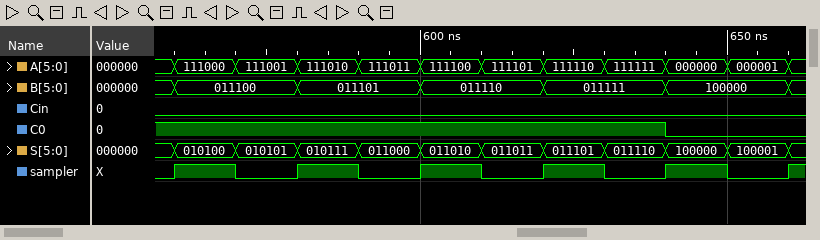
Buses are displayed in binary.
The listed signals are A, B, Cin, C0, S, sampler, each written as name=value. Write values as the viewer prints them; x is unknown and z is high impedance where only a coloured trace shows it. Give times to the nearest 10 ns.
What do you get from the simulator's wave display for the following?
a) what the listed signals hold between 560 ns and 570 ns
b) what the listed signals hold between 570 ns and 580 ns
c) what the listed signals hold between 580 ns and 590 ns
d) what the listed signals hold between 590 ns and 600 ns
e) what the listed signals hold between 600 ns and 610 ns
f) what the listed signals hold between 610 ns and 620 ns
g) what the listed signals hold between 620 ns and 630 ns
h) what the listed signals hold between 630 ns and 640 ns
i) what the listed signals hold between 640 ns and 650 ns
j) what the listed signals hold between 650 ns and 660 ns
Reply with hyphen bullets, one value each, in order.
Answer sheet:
- A=111000, B=011100, Cin=0, C0=1, S=010100, sampler=1
- A=111001, B=011100, Cin=0, C0=1, S=010101, sampler=0
- A=111010, B=011101, Cin=0, C0=1, S=010111, sampler=1
- A=111011, B=011101, Cin=0, C0=1, S=011000, sampler=0
- A=111100, B=011110, Cin=0, C0=1, S=011010, sampler=1
- A=111101, B=011110, Cin=0, C0=1, S=011011, sampler=0
- A=111110, B=011111, Cin=0, C0=1, S=011101, sampler=1
- A=111111, B=011111, Cin=0, C0=1, S=011110, sampler=0
- A=000000, B=100000, Cin=0, C0=0, S=100000, sampler=1
- A=000001, B=100000, Cin=0, C0=0, S=100001, sampler=0
